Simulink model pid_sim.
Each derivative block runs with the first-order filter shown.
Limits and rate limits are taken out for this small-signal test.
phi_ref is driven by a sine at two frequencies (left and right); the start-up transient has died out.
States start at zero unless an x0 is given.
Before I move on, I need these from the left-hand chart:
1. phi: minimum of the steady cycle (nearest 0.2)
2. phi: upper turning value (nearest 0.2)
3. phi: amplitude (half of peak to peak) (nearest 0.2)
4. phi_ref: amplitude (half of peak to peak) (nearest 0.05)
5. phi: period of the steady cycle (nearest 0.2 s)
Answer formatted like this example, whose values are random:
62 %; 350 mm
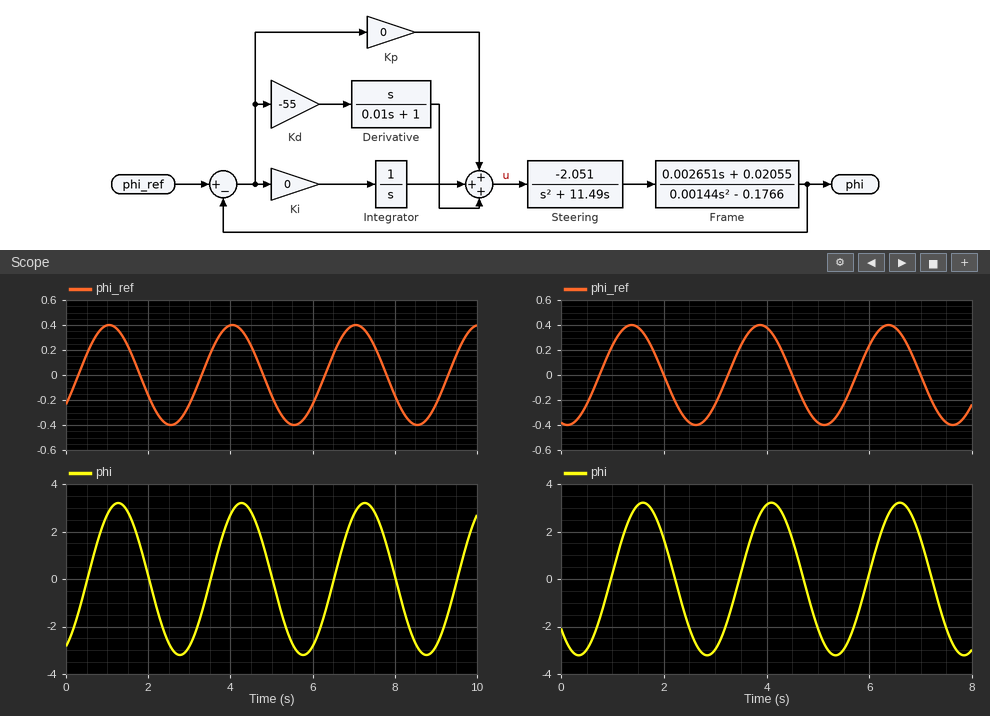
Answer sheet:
-3.2; 3.2; 3.2; 0.40; 3.0 s
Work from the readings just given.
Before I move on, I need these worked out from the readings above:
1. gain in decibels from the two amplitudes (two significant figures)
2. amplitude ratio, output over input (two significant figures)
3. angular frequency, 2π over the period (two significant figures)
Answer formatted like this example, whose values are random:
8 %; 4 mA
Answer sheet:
18 dB; 8.0; 2.1 rad/s
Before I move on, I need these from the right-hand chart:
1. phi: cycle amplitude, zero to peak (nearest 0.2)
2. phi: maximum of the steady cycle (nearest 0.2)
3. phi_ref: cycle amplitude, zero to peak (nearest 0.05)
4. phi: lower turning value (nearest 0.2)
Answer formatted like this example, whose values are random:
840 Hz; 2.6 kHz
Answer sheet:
3.2; 3.2; 0.40; -3.2
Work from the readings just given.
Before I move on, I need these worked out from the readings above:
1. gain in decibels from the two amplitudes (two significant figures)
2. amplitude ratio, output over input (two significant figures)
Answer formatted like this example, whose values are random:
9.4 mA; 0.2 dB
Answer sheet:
18 dB; 8.0
